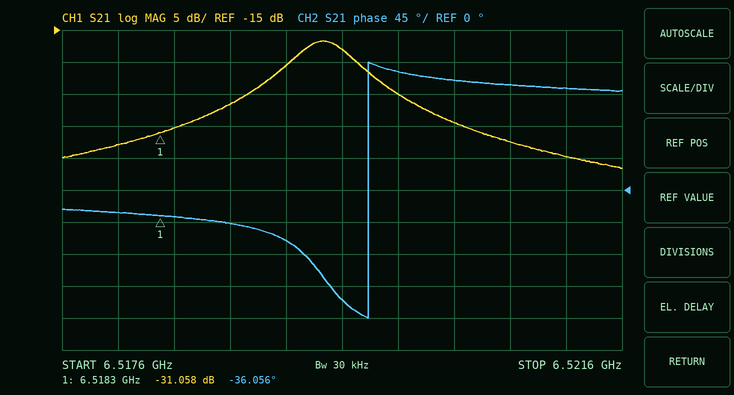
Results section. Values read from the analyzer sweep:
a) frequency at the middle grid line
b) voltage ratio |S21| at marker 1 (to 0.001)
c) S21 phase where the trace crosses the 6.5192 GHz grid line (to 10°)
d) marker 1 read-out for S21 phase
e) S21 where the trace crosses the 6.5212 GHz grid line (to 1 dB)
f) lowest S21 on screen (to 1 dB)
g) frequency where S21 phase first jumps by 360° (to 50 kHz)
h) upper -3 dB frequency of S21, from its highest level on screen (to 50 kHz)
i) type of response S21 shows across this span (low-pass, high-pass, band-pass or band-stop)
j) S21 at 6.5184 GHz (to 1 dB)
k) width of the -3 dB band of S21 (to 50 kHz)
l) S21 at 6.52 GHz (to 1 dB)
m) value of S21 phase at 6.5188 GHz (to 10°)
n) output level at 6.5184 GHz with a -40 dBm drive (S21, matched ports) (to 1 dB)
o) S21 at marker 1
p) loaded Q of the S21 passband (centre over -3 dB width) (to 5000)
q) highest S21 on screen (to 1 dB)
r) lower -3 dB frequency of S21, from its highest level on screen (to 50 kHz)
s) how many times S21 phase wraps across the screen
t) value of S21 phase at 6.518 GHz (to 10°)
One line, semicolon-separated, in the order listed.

6.5196 GHz; 0.028; -70°; -36.056°; -35 dB; -37 dB; 6.51980 GHz; 6.51970 GHz; band-pass; -30 dB; 450 kHz; -25 dB; -50°; -70 dBm; -31.058 dB; 15000; -17 dB; 6.51925 GHz; 1; -30°
